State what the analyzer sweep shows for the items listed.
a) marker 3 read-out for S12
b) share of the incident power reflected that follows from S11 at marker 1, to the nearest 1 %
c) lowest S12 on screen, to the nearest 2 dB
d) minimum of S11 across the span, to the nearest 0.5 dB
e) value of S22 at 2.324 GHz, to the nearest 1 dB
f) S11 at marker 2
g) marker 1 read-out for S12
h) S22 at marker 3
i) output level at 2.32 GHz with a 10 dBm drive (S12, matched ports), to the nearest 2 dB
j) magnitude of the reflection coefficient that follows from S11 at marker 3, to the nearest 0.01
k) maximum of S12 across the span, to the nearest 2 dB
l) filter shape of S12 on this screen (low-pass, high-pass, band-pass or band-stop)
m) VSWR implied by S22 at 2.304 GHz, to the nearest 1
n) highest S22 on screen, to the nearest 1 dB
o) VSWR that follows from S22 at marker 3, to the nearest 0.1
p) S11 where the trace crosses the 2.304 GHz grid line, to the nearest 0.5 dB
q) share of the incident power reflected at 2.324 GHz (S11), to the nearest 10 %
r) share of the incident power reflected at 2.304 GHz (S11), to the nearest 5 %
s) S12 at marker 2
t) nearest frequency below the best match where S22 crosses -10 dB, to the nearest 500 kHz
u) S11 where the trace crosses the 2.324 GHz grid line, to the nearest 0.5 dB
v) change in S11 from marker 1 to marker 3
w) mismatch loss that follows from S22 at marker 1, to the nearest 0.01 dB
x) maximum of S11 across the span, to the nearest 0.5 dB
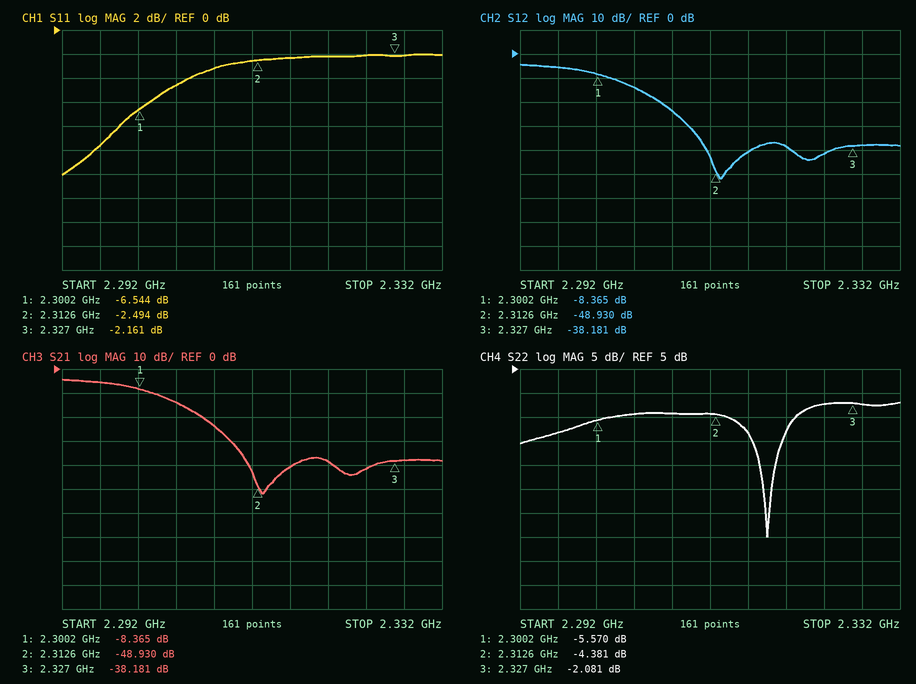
-38.181 dB
22 %
-52 dB
-12.0 dB
-2 dB
-2.494 dB
-8.365 dB
-2.081 dB
-28 dBm
0.78
-4 dB
low-pass
4
-2 dB
8.4
-4.5 dB
60 %
35 %
-48.930 dB
2.3165 GHz
-2.0 dB
4.383 dB
1.41 dB
-2.0 dB
